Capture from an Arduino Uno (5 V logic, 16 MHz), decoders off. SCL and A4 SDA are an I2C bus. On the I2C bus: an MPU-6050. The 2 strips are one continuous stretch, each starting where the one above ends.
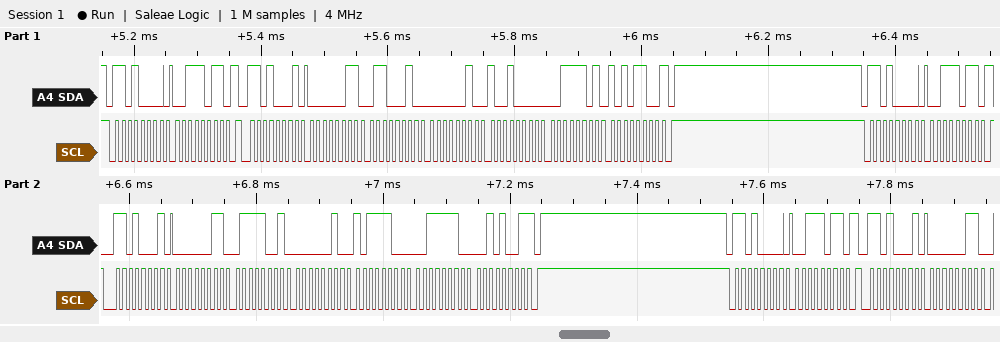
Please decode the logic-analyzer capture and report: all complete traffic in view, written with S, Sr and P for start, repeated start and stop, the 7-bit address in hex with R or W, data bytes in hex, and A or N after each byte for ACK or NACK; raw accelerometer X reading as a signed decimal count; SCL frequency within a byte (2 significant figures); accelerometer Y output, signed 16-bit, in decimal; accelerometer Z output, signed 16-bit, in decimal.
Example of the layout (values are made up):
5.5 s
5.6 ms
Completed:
S 68W A 3B A Sr 68R A 03 A 62 A 02 A 90 A 3D A AC N P S 68W A 3B A Sr 68R A 03 A 79 A 02 A BC A 3E A 29 N P S 68W A 3B A Sr 68R A 03 A
866
100 kHz
656
15788
